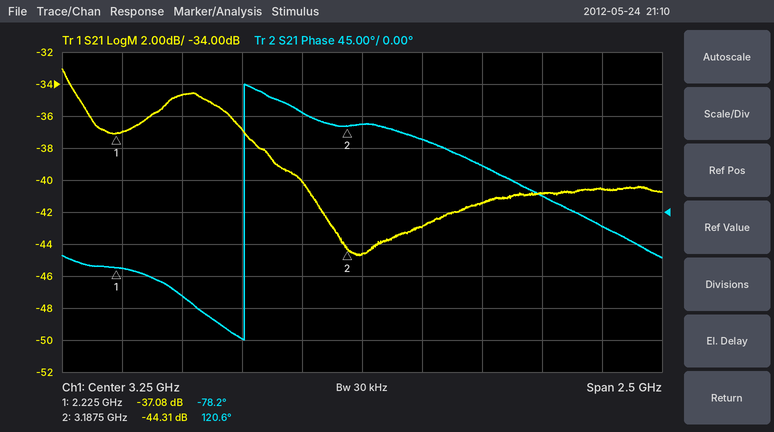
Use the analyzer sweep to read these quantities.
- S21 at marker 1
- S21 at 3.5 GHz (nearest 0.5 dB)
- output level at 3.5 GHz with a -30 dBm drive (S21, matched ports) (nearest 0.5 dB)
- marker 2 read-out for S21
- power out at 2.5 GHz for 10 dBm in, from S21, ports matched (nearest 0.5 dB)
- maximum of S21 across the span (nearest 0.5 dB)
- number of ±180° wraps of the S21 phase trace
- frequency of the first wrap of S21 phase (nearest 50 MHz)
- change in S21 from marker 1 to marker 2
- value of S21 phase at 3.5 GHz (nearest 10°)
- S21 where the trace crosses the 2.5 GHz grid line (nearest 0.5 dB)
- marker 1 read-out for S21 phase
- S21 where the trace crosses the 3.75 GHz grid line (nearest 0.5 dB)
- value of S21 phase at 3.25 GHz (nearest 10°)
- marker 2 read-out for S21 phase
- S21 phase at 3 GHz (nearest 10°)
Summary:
-37.08 dB
-43.0 dB
-73.0 dBm
-44.31 dB
-24.5 dBm
-33.0 dB
1
2.75 GHz
-7.23 dB
100°
-34.5 dB
-78.2°
-41.5 dB
120°
120.6°
140°
